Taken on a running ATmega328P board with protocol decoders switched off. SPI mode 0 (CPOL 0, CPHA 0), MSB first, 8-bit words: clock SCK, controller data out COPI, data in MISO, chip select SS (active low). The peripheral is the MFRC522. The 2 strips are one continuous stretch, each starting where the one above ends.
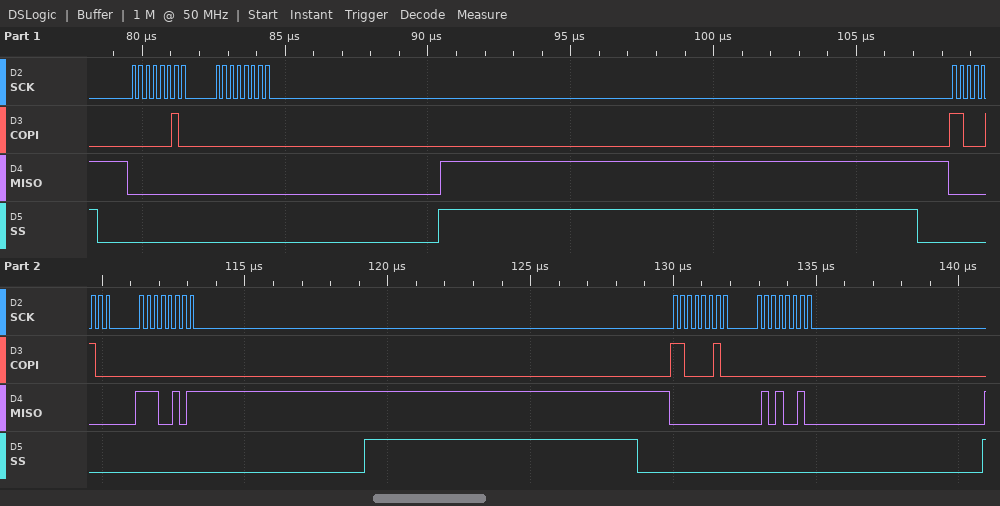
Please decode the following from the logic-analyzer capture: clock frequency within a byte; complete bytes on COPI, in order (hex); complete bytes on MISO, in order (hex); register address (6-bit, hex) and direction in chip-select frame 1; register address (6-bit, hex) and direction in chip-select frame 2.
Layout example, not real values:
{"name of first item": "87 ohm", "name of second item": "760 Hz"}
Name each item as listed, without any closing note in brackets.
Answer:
{"clock frequency within a byte": "4 MHz", "complete bytes on COPI, in order": "0x02 0x00 0xC4 0x00 0xC2 0x00", "complete bytes on MISO, in order": "0x00 0x00 0x00 0xE5 0x00 0x52", "register address (6-bit, hex) and direction in chip-select frame 1": "0x01 write", "register address (6-bit, hex) and direction in chip-select frame 2": "0x22 read"}
